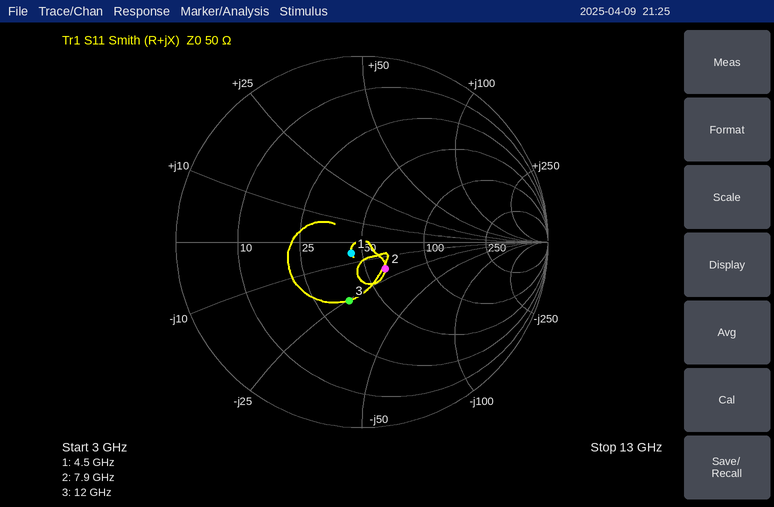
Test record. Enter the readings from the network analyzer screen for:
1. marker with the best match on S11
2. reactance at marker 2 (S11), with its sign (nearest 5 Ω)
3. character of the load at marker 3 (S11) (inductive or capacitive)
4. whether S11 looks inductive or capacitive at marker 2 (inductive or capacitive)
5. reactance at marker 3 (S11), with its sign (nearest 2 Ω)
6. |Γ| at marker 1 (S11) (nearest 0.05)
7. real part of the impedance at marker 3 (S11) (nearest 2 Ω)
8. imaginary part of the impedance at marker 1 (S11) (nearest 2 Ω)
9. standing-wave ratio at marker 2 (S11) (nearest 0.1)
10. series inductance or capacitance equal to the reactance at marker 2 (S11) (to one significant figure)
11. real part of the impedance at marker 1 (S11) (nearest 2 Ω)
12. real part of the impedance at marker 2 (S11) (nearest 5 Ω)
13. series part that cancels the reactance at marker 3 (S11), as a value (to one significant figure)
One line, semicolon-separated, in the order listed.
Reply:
marker 1; -20 Ω; capacitive; capacitive; -26 Ω; 0.10; 36 Ω; -6 Ω; 1.5; 1 pF; 44 Ω; 60 Ω; 300 pH
